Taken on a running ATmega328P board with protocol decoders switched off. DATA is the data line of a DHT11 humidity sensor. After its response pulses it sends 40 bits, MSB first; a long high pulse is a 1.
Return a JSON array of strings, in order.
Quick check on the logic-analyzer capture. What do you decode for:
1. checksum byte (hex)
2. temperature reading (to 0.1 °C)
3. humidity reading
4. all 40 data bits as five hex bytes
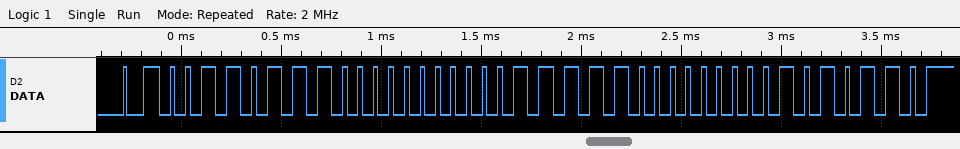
["0x56", "31.0 °C", "55 %", "37 00 1F 00 56"]
